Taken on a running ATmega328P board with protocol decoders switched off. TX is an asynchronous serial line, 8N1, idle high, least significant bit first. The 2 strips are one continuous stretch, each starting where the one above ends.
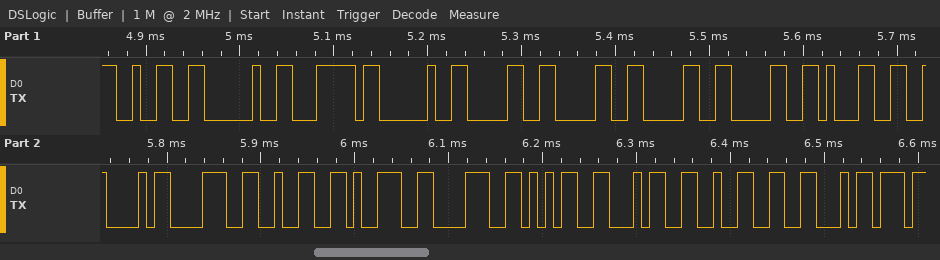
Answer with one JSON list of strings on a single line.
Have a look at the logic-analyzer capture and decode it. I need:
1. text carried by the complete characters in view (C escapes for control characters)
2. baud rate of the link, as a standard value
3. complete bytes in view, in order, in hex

["\"2 | 00001B8298542F\"", "115200 baud", "32 20 7C 20 30 30 30 30 31 42 38 32 39 38 35 34 32 46"]
